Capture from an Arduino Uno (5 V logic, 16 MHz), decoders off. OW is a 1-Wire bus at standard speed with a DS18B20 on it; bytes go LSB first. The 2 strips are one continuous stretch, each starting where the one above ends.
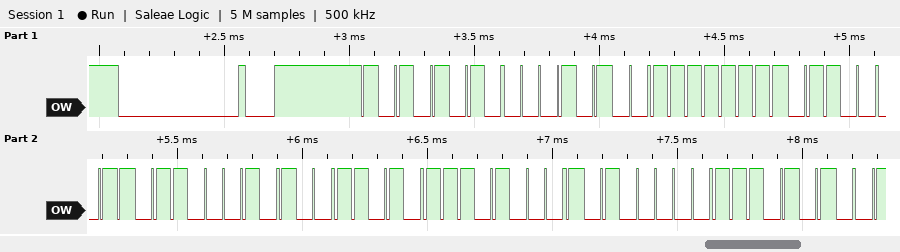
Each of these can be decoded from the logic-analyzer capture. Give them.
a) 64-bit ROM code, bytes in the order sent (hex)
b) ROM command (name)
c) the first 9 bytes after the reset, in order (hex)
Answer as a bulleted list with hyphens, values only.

- 28 FF C6 46 59 17 05 57
- Match ROM
- 55 28 FF C6 46 59 17 05 57
